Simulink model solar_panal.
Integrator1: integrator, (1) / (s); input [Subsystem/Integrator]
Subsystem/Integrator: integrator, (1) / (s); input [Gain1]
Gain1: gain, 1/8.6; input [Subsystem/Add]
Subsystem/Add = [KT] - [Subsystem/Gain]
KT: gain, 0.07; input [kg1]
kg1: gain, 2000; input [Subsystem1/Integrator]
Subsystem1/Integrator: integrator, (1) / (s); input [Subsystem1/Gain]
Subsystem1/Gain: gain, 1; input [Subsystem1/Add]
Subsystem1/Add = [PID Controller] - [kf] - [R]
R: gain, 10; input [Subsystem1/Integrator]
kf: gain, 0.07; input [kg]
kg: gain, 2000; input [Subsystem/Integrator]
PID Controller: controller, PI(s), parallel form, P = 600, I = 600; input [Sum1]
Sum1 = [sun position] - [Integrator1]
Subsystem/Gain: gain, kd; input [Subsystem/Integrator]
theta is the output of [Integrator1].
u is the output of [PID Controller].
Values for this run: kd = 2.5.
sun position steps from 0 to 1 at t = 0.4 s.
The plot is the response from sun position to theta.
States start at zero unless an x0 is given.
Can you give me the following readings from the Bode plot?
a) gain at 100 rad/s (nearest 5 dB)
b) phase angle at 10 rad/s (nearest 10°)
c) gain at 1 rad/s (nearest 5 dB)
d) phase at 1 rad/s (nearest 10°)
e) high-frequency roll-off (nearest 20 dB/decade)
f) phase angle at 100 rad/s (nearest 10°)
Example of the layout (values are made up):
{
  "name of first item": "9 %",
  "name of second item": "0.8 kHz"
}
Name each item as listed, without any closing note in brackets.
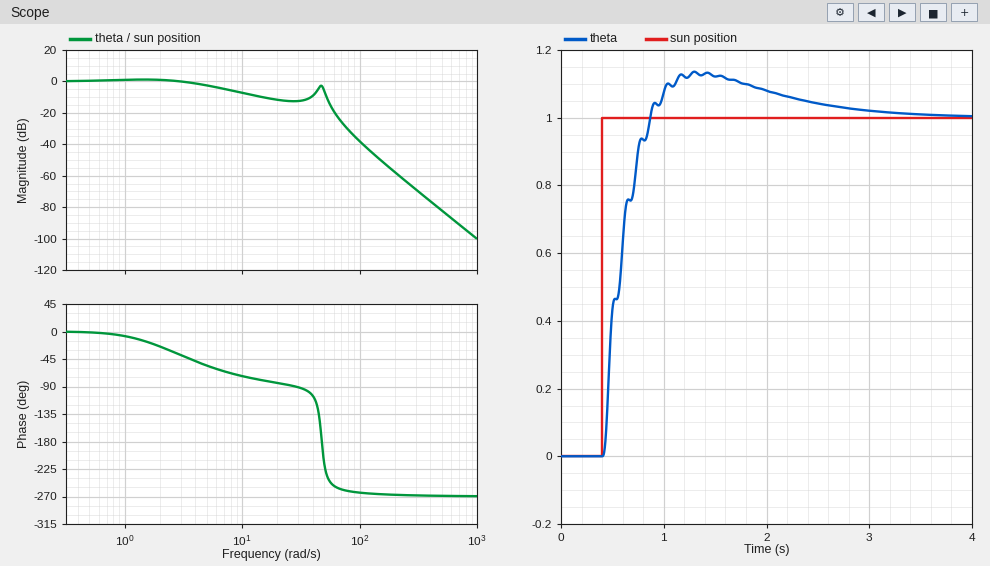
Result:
{
  "gain at 100 rad/s": "-40 dB",
  "phase angle at 10 rad/s": "-70°",
  "gain at 1 rad/s": "0 dB",
  "phase at 1 rad/s": "-10°",
  "high-frequency roll-off": "-60 dB/decade",
  "phase angle at 100 rad/s": "-260°"
}
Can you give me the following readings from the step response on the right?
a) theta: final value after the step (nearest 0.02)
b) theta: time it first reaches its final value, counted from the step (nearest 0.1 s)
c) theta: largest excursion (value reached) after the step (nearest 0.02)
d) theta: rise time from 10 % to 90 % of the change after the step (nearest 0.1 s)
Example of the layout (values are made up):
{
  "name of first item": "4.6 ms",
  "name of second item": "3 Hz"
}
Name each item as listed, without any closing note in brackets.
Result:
{
  "theta: final value after the step": "1.00",
  "theta: time it first reaches its final value, counted from the step": "0.5 s",
  "theta: largest excursion (value reached) after the step": "1.14",
  "theta: rise time from 10 % to 90 % of the change after the step": "0.3 s"
}
